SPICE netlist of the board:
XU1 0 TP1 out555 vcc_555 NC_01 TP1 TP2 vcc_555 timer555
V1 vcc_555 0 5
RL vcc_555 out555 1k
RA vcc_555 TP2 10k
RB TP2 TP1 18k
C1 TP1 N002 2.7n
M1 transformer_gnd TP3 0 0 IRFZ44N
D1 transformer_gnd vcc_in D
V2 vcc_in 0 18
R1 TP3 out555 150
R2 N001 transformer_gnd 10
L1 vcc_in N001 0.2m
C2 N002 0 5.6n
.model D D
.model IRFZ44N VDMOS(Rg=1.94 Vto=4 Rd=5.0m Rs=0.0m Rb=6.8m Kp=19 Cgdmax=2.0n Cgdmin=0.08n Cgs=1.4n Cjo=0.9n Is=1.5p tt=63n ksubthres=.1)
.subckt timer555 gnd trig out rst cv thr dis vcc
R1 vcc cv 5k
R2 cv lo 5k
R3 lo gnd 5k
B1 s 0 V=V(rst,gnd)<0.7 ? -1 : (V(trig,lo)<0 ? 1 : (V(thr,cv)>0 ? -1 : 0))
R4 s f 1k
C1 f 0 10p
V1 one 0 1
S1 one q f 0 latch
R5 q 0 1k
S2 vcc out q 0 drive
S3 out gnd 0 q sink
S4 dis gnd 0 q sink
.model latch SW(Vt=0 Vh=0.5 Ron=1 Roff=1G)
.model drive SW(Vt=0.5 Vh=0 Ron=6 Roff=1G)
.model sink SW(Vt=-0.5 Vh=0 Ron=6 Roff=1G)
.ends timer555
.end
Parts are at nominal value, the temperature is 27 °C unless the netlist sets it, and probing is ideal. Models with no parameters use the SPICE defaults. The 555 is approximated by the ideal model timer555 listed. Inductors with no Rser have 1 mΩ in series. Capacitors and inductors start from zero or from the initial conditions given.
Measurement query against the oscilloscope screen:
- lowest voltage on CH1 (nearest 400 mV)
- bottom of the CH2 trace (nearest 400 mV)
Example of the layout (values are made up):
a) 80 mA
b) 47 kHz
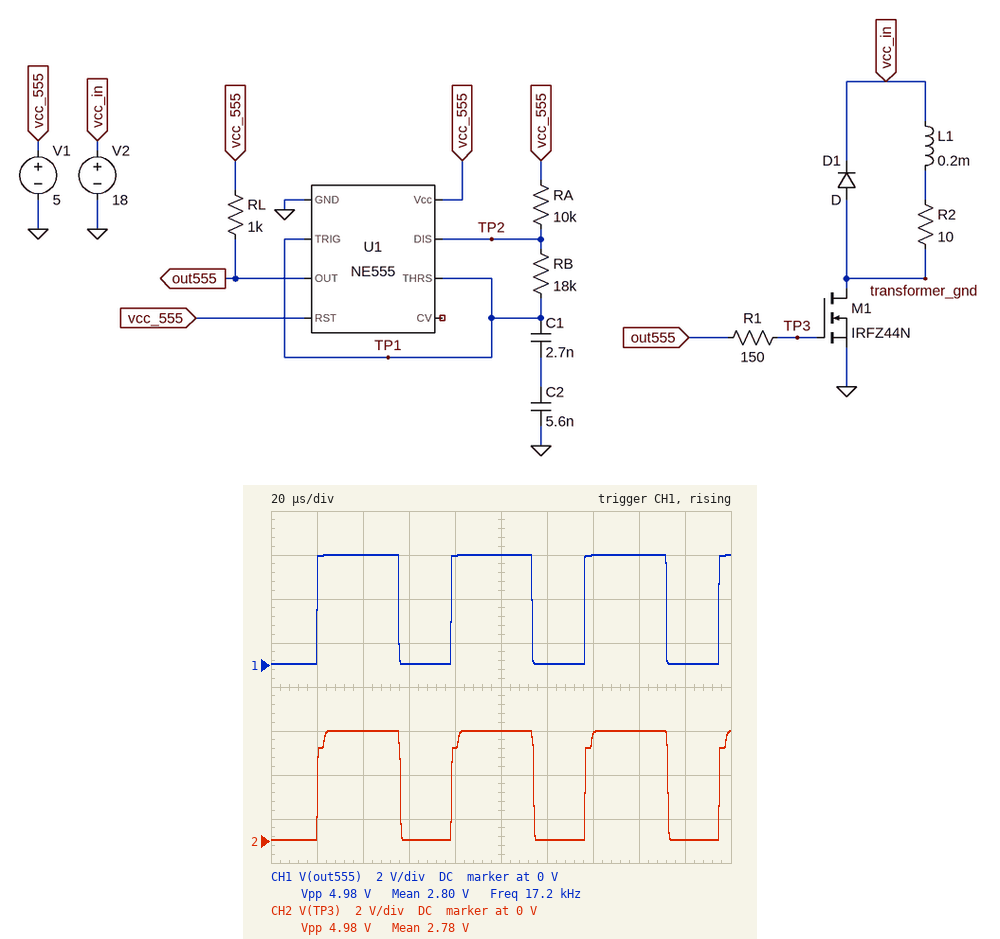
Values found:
a) 0 V
b) 0 V
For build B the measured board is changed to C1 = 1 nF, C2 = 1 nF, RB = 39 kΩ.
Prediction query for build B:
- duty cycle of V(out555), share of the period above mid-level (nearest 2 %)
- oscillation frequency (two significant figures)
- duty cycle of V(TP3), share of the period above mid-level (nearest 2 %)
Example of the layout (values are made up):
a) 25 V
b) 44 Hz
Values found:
a) 56 %
b) 33 kHz
c) 58 %
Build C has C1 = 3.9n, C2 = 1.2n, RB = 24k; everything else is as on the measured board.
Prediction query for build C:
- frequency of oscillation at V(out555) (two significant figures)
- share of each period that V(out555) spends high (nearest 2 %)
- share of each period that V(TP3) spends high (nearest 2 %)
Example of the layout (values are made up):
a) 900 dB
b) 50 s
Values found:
a) 27 kHz
b) 58 %
c) 60 %
